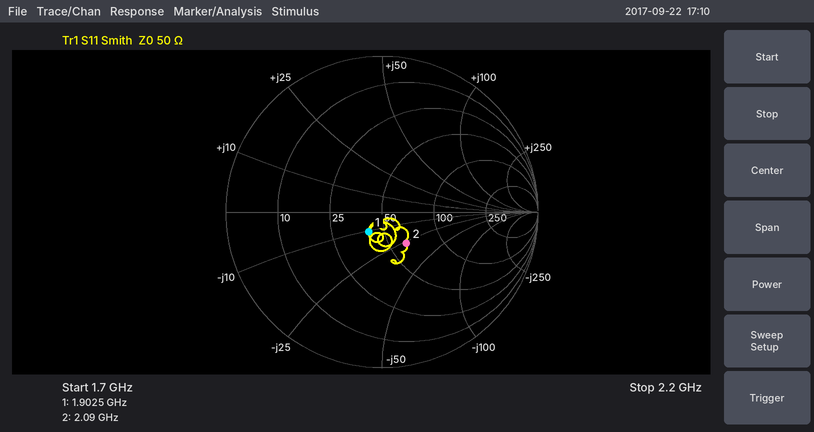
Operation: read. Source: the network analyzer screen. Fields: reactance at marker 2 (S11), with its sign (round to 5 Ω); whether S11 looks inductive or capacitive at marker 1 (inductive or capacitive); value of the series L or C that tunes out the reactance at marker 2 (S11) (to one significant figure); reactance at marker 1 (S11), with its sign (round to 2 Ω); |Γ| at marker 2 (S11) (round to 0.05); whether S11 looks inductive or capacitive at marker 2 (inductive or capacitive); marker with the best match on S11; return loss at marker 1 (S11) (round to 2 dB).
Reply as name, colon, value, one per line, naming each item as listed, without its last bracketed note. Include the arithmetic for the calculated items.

reactance at marker 2 (S11), with its sign: -25 Ω
whether S11 looks inductive or capacitive at marker 1: capacitive
value of the series L or C that tunes out the reactance at marker 2 (S11): L = 25 Ω/(2π × 2.09 GHz) ≈ 2 nH
reactance at marker 1 (S11), with its sign: -10 Ω
|Γ| at marker 2 (S11): 0.25
whether S11 looks inductive or capacitive at marker 2: capacitive
marker with the best match on S11: marker 1
return loss at marker 1 (S11): 16 dB
